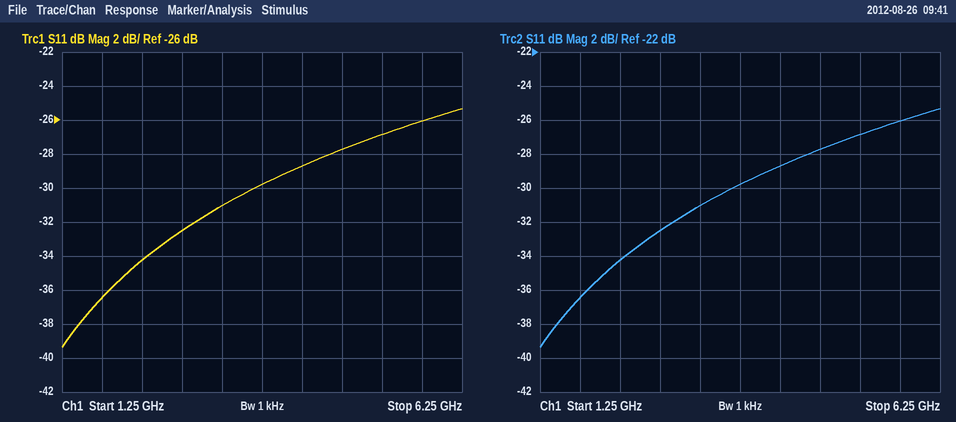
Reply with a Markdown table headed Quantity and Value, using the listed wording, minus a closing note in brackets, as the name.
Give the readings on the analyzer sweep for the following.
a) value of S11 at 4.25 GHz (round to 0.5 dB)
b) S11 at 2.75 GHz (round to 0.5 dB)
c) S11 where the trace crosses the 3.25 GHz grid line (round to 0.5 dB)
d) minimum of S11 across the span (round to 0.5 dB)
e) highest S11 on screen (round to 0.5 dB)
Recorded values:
| Quantity | Value |
|---|---|
| value of S11 at 4.25 GHz | -28.5 dB |
| S11 at 2.75 GHz | -32.5 dB |
| S11 where the trace crosses the 3.25 GHz grid line | -31.0 dB |
| minimum of S11 across the span | -39.5 dB |
| highest S11 on screen | -25.5 dB |
